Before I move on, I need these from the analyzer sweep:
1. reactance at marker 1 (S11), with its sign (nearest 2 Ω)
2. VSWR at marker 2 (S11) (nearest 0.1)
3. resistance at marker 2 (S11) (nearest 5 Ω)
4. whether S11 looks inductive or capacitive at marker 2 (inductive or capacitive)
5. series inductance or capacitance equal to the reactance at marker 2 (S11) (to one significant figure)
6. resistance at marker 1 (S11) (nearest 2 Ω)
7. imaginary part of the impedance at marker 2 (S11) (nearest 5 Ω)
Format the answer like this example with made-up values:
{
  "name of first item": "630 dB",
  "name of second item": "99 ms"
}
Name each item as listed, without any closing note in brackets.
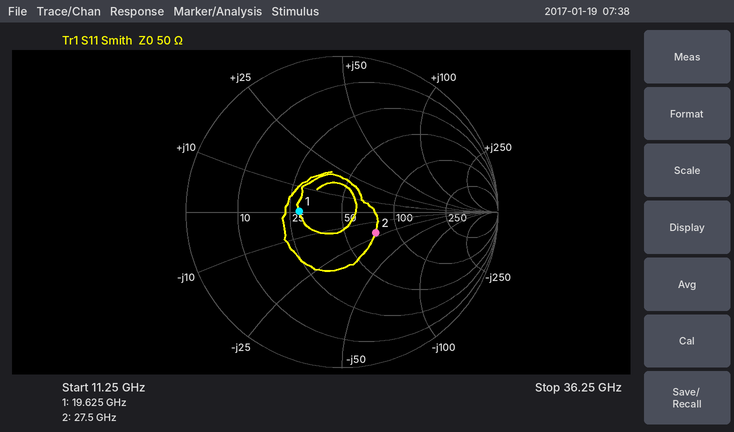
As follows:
{
  "reactance at marker 1 (S11), with its sign": "0 Ω",
  "VSWR at marker 2 (S11)": "1.7",
  "resistance at marker 2 (S11)": "75 Ω",
  "whether S11 looks inductive or capacitive at marker 2": "capacitive",
  "series inductance or capacitance equal to the reactance at marker 2 (S11)": "300 fF",
  "resistance at marker 1 (S11)": "28 Ω",
  "imaginary part of the impedance at marker 2 (S11)": "-20 Ω"
}
